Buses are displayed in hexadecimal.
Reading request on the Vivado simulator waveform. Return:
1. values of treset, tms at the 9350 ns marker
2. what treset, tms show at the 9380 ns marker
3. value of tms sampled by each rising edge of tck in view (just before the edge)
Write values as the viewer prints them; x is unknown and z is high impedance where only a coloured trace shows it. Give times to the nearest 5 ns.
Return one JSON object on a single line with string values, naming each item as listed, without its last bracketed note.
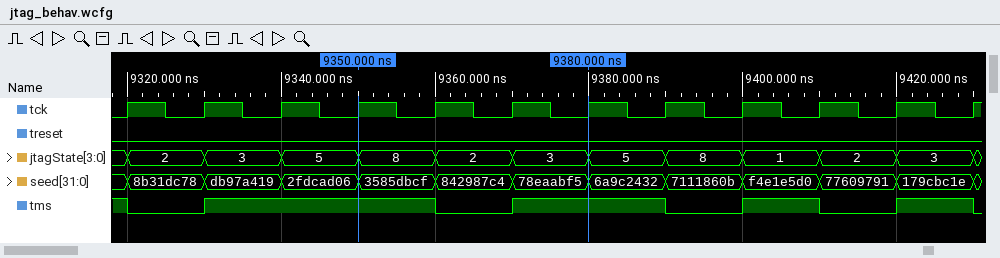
{"values of treset, tms at the 9350 ns marker": "treset=0, tms=1", "what treset, tms show at the 9380 ns marker": "treset=0, tms=1", "value of tms sampled by each rising edge of tck in view": "1 0 1 1 1 0 1 1 0 1 0 1"}
